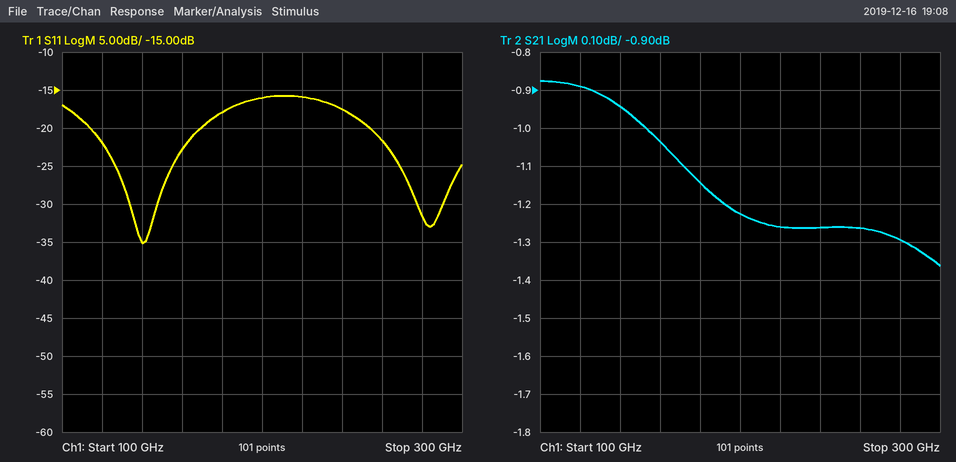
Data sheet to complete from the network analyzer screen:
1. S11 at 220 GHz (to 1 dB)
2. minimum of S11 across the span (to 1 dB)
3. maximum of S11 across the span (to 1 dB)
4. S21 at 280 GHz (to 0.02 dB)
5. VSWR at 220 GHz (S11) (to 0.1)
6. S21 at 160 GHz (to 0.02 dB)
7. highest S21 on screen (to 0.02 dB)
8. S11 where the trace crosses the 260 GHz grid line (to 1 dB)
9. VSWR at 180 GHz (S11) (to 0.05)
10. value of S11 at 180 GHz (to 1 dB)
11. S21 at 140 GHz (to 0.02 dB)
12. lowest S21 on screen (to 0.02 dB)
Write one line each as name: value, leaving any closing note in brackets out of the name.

S11 at 220 GHz: -16 dB
minimum of S11 across the span: -35 dB
maximum of S11 across the span: -16 dB
S21 at 280 GHz: -1.30 dB
VSWR at 220 GHz (S11): 1.4
S21 at 160 GHz: -1.04 dB
highest S21 on screen: -0.88 dB
S11 where the trace crosses the 260 GHz grid line: -22 dB
VSWR at 180 GHz (S11): 1.30
value of S11 at 180 GHz: -18 dB
S21 at 140 GHz: -0.94 dB
lowest S21 on screen: -1.36 dB
